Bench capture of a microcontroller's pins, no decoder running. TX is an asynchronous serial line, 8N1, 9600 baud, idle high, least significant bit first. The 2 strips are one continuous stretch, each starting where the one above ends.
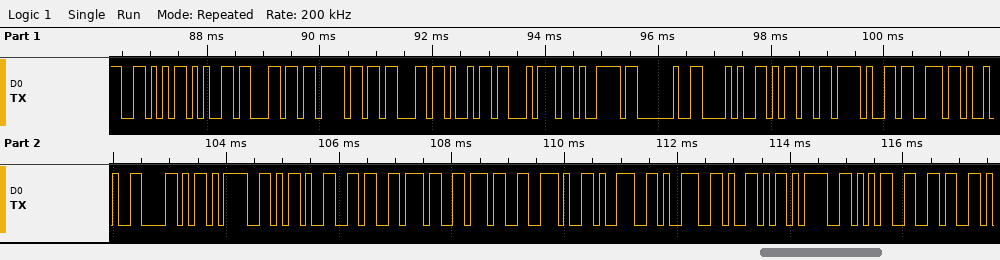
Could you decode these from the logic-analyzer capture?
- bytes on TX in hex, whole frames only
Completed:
0x56 0x65 0x6C 0x6F 0x63 0x69 0x74 0x79 0x20 0x28 0x6D 0x2F 0x73 0x29 0x58 0x3D 0x2D 0x36 0x37 0x37 0x2E 0x39 0x39 0x59 0x3D 0x35 0x36
